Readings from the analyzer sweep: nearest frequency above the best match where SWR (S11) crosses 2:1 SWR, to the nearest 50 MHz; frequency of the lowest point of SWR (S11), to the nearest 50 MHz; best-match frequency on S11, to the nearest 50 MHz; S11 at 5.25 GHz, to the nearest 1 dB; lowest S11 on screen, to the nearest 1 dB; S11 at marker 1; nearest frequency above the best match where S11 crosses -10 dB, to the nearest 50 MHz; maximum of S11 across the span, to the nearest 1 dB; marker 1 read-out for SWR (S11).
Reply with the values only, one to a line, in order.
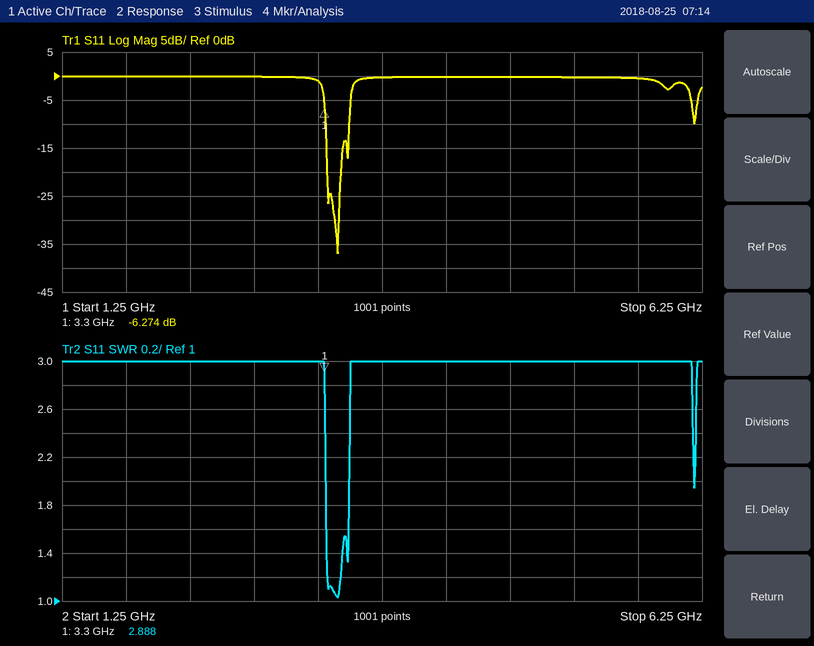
3.50 GHz
3.40 GHz
3.40 GHz
0 dB
-37 dB
-6.274 dB
3.50 GHz
0 dB
2.888
